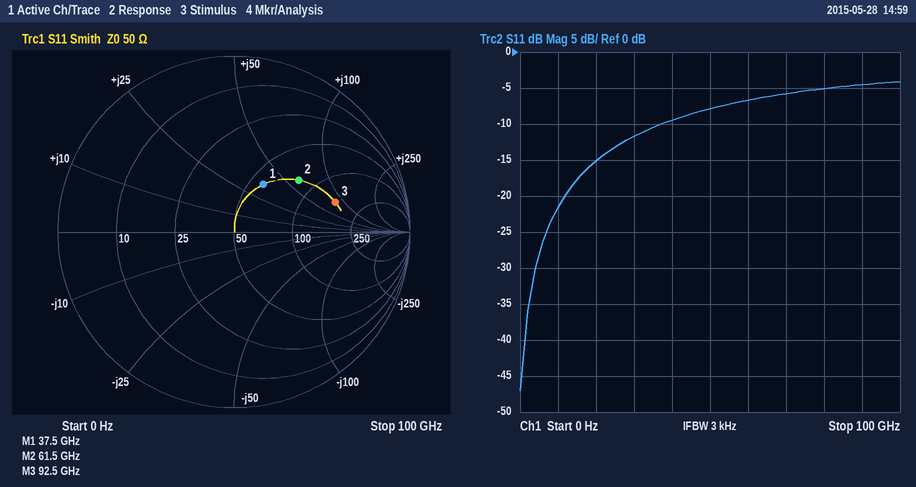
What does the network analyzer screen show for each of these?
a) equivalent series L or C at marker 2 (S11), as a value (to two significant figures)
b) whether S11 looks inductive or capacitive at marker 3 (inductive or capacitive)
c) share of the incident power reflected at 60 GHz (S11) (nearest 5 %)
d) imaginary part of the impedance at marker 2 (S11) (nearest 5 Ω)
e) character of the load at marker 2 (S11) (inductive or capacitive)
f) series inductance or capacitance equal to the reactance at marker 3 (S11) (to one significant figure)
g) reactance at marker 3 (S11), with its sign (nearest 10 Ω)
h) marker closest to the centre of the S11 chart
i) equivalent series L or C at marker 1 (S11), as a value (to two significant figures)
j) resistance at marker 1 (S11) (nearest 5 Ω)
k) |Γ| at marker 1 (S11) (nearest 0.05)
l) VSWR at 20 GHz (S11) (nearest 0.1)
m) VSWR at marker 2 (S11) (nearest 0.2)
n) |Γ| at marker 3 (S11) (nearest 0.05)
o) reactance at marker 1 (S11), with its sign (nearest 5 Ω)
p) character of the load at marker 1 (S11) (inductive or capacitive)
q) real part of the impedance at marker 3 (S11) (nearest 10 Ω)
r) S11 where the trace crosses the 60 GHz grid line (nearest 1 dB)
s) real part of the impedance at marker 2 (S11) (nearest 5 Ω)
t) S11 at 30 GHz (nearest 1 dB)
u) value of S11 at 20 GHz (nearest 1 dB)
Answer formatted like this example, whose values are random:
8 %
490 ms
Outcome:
160 pH
inductive
20 %
+60 Ω
inductive
100 pH
+80 Ω
marker 1
150 pH
60 Ω
0.30
1.4
2.8
0.60
+35 Ω
inductive
150 Ω
-7 dB
80 Ω
-12 dB
-15 dB
